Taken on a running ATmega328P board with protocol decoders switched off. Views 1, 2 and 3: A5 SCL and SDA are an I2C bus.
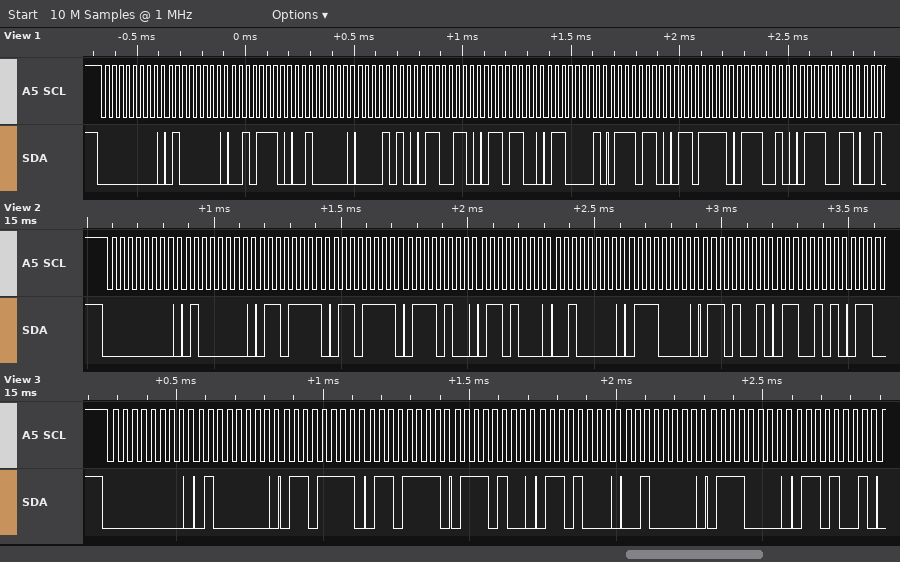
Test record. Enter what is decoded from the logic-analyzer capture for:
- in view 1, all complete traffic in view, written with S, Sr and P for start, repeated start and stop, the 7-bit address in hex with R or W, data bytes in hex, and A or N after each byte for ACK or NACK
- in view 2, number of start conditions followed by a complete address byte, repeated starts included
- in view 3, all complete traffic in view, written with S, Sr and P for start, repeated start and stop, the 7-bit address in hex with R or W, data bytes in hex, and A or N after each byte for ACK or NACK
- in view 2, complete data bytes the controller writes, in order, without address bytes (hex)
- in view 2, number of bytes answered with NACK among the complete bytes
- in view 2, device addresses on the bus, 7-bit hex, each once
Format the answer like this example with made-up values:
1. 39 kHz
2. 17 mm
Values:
1. S 00W A 40 A 2E A 20 A 0A A 66 A 6C A 61 A 76 A 6F A 72 A 73 A
2. 1
3. S 00W A 40 A 6F A 6F A 74 A 68 A 20 A 70 A 69 A
4. 40 6F 6F 74 68 20 70 69 65
5. 0
6. 0x00
